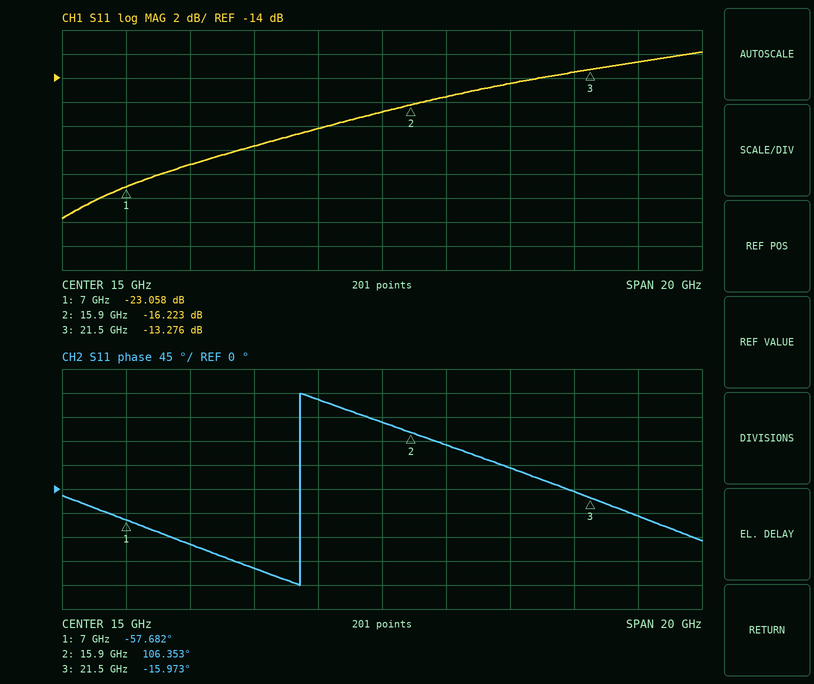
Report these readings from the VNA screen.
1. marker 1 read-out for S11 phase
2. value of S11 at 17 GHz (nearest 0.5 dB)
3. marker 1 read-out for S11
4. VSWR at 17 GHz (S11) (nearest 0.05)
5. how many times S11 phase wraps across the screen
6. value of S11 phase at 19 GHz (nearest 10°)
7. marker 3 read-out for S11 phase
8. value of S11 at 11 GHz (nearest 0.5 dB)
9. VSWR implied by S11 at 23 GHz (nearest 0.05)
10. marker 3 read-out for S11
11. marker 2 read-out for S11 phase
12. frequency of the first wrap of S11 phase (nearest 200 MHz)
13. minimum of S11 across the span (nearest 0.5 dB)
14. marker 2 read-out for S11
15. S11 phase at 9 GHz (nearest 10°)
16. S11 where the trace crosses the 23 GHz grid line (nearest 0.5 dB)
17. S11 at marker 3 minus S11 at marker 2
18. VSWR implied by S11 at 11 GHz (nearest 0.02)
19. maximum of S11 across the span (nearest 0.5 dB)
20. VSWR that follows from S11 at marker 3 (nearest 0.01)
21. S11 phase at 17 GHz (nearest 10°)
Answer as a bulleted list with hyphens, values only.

- -57.682°
- -15.5 dB
- -23.058 dB
- 1.40
- 1
- 40°
- -15.973°
- -19.5 dB
- 1.60
- -13.276 dB
- 106.353°
- 12.4 GHz
- -25.5 dB
- -16.223 dB
- -100°
- -12.5 dB
- 2.947 dB
- 1.24
- -12.0 dB
- 1.55
- 80°
